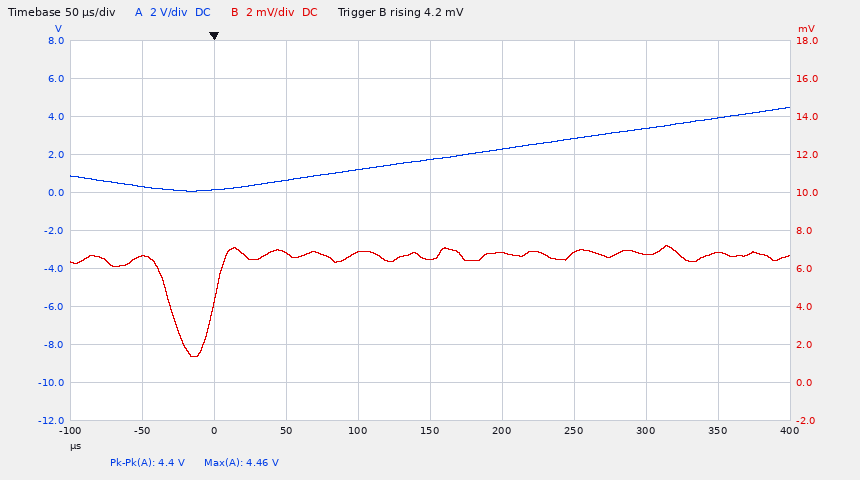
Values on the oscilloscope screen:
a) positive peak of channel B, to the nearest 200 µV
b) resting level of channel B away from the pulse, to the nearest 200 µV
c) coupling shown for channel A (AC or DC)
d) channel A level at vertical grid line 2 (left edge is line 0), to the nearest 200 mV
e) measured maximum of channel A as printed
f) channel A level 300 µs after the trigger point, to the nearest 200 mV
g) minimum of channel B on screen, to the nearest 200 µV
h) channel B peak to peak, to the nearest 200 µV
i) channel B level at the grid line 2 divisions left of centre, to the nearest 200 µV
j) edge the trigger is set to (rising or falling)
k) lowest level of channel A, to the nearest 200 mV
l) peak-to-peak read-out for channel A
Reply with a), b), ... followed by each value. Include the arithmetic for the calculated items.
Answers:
a) 7.2 mV
b) 6.6 mV
c) DC
d) 200 mV
e) 4.46 V
f) 3.4 V
g) 1.4 mV
h) 7.2 mV − (1.4 mV) = 5.8 mV
i) 6.8 mV
j) rising
k) 0.0 V
l) 4.4 V
